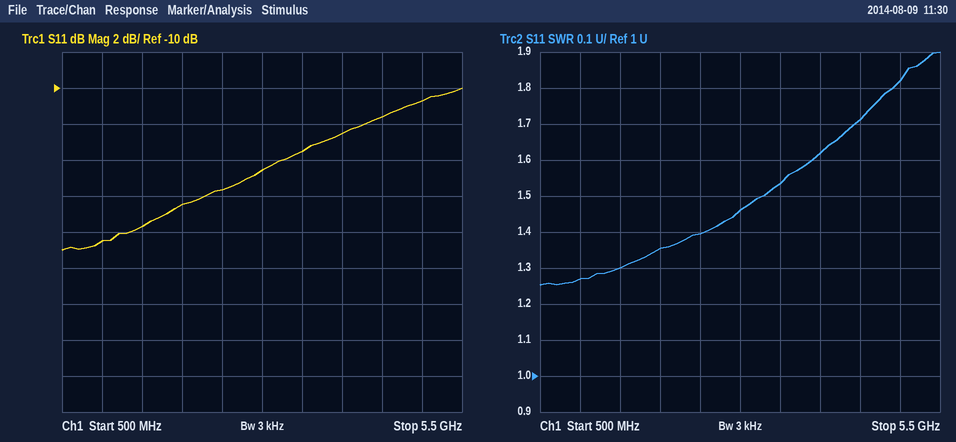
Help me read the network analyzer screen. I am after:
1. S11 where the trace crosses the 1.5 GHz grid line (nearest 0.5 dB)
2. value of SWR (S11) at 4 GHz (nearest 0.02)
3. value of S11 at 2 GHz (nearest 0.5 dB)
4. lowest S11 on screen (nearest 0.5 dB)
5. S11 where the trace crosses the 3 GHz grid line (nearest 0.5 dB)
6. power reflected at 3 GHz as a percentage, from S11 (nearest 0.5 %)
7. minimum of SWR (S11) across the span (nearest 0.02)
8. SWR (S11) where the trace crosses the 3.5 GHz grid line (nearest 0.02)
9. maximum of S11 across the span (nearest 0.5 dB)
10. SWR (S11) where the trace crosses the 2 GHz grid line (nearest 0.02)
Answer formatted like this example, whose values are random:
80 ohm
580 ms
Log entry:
-17.5 dB
1.62
-16.5 dB
-19.0 dB
-14.5 dB
3.5 %
1.26
1.54
-10.0 dB
1.36
